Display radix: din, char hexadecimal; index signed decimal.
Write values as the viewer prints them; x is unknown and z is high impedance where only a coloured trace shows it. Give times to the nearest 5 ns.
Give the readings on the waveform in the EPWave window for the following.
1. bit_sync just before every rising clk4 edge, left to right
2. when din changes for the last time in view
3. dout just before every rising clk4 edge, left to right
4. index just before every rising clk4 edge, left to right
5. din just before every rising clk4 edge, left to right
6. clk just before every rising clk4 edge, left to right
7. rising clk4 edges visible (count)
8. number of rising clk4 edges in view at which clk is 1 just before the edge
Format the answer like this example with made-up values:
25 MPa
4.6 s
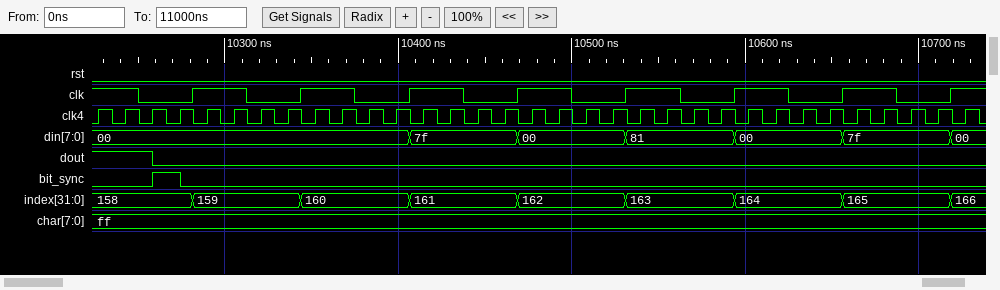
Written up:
0 0 0 1 0 0 0 0 0 0 0 0 0 0 0 0 0 0 0 0 0 0 0 0 0 0 0 0 0 0 0 0 0
10720 ns
1 1 1 0 0 0 0 0 0 0 0 0 0 0 0 0 0 0 0 0 0 0 0 0 0 0 0 0 0 0 0 0 0
158, 158, 158, 158, 159, 159, 159, 159, 160, 160, 160, 160, 161, 161, 161, 161, 162, 162, 162, 162, 163, 163, 163, 163, 164, 164, 164, 164, 165, 165, 165, 165, 166
00, 00, 00, 00, 00, 00, 00, 00, 00, 00, 00, 00, 7f, 7f, 7f, 7f, 00, 00, 00, 00, 81, 81, 81, 81, 00, 00, 00, 00, 7f, 7f, 7f, 7f, 00
1 1 0 0 1 1 0 0 1 1 0 0 1 1 0 0 1 1 0 0 1 1 0 0 1 1 0 0 1 1 0 0 1
33
17
